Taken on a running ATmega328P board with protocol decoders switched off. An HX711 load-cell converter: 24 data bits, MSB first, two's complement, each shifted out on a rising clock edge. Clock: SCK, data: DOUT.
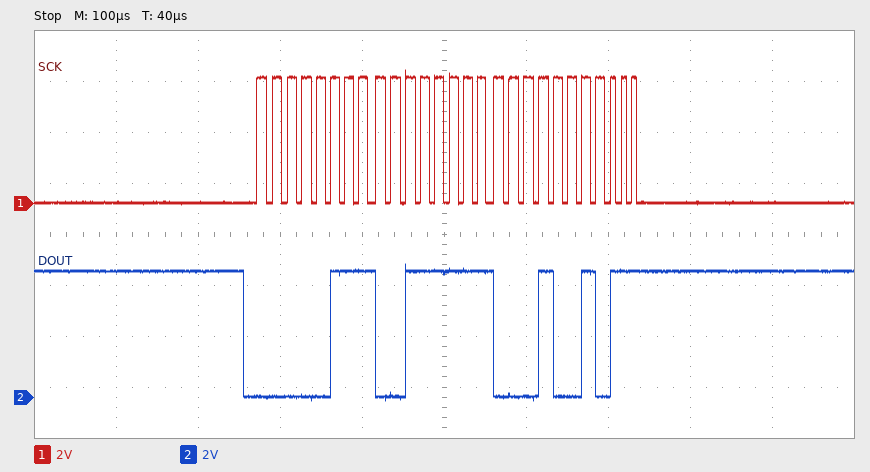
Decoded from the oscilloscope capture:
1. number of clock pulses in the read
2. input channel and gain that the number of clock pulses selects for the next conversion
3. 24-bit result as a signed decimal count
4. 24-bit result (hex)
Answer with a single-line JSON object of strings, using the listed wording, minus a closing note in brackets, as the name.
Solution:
{"number of clock pulses in the read": "27", "input channel and gain that the number of clock pulses selects for the next conversion": "channel A, gain 64", "24-bit result as a signed decimal count": "474898", "24-bit result": "0x073F12"}
